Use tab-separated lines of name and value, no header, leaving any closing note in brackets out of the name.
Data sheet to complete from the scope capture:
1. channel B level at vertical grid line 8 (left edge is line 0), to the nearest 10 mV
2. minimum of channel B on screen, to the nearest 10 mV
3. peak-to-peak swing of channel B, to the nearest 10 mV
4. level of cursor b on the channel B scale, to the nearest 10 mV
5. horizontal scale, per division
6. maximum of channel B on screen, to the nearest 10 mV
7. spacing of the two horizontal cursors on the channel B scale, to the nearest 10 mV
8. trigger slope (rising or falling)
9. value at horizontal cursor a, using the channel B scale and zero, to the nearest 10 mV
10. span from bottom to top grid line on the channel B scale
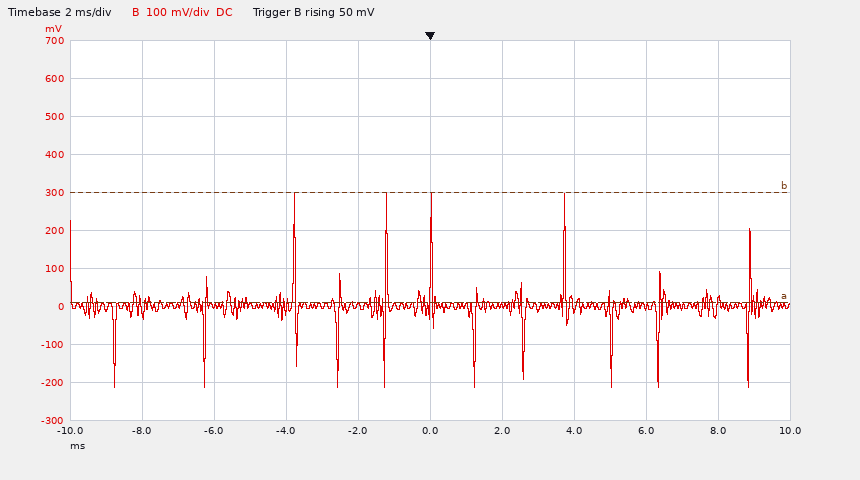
channel B level at vertical grid line 8 (left edge is line 0), to the nearest 10 mV	0 mV
minimum of channel B on screen, to the nearest 10 mV	-210 mV
peak-to-peak swing of channel B, to the nearest 10 mV	510 mV
level of cursor b on the channel B scale, to the nearest 10 mV	300 mV
horizontal scale, per division	2 ms
maximum of channel B on screen, to the nearest 10 mV	300 mV
spacing of the two horizontal cursors on the channel B scale, to the nearest 10 mV	290 mV
trigger slope	rising
value at horizontal cursor a, using the channel B scale and zero, to the nearest 10 mV	10 mV
span from bottom to top grid line on the channel B scale	1 V
